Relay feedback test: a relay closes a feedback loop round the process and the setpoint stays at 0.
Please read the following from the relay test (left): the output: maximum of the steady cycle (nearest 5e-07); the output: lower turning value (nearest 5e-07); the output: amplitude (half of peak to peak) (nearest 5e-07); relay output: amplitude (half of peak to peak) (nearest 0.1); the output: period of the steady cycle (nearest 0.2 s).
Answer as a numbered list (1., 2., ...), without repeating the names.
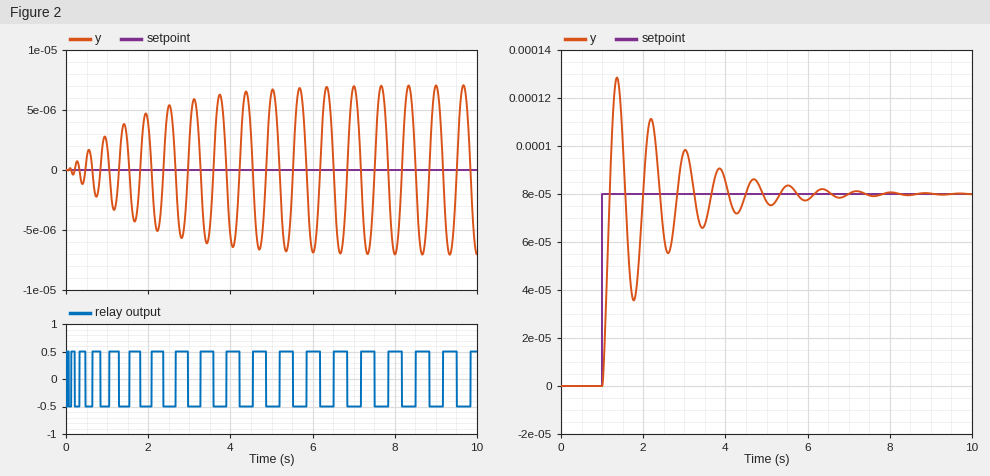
1. 0.0000070
2. -0.0000070
3. 0.0000070
4. 0.5
5. 0.6 s
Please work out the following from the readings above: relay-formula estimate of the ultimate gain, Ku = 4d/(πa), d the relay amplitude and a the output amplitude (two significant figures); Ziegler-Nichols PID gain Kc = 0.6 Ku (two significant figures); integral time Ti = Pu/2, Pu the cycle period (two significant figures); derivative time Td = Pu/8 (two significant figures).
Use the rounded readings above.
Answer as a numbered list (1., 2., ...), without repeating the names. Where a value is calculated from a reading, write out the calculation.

1. 4 × 0.5 / (π × 7e-06) = 91000
2. 0.6 × 91000 = 55000
3. 0.6 / 2 = 0.30 s
4. 0.6 / 8 = 0.075 s
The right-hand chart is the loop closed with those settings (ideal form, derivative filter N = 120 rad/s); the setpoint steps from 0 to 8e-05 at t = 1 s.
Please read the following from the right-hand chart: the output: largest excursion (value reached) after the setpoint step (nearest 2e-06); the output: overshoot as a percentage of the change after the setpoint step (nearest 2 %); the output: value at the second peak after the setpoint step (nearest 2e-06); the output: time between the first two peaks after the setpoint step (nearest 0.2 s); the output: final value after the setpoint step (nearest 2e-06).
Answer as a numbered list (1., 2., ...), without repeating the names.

1. 0.000128
2. 60 %
3. 0.000112
4. 0.8 s
5. 0.000080
